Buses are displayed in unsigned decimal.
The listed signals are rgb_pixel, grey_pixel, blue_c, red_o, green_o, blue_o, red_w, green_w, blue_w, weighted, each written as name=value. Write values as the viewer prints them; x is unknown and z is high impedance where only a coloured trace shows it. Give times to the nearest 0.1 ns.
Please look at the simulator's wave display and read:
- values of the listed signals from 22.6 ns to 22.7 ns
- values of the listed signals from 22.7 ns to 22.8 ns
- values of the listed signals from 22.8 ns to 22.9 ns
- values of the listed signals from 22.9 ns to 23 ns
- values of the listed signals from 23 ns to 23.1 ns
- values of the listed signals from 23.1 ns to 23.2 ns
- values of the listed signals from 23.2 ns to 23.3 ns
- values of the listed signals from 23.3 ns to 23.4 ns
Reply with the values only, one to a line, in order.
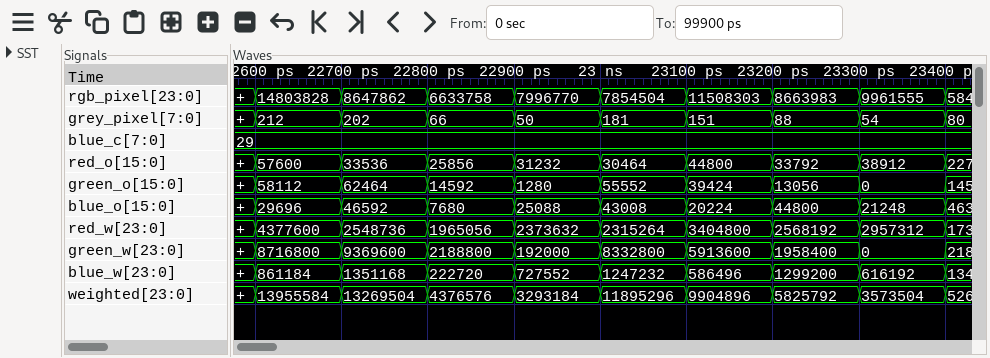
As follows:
rgb_pixel=14803828, grey_pixel=212, blue_c=29, red_o=57600, green_o=58112, blue_o=29696, red_w=4377600, green_w=8716800, blue_w=861184, weighted=13955584
rgb_pixel=8647862, grey_pixel=202, blue_c=29, red_o=33536, green_o=62464, blue_o=46592, red_w=2548736, green_w=9369600, blue_w=1351168, weighted=13269504
rgb_pixel=6633758, grey_pixel=66, blue_c=29, red_o=25856, green_o=14592, blue_o=7680, red_w=1965056, green_w=2188800, blue_w=222720, weighted=4376576
rgb_pixel=7996770, grey_pixel=50, blue_c=29, red_o=31232, green_o=1280, blue_o=25088, red_w=2373632, green_w=192000, blue_w=727552, weighted=3293184
rgb_pixel=7854504, grey_pixel=181, blue_c=29, red_o=30464, green_o=55552, blue_o=43008, red_w=2315264, green_w=8332800, blue_w=1247232, weighted=11895296
rgb_pixel=11508303, grey_pixel=151, blue_c=29, red_o=44800, green_o=39424, blue_o=20224, red_w=3404800, green_w=5913600, blue_w=586496, weighted=9904896
rgb_pixel=8663983, grey_pixel=88, blue_c=29, red_o=33792, green_o=13056, blue_o=44800, red_w=2568192, green_w=1958400, blue_w=1299200, weighted=5825792
rgb_pixel=9961555, grey_pixel=54, blue_c=29, red_o=38912, green_o=0, blue_o=21248, red_w=2957312, green_w=0, blue_w=616192, weighted=3573504
